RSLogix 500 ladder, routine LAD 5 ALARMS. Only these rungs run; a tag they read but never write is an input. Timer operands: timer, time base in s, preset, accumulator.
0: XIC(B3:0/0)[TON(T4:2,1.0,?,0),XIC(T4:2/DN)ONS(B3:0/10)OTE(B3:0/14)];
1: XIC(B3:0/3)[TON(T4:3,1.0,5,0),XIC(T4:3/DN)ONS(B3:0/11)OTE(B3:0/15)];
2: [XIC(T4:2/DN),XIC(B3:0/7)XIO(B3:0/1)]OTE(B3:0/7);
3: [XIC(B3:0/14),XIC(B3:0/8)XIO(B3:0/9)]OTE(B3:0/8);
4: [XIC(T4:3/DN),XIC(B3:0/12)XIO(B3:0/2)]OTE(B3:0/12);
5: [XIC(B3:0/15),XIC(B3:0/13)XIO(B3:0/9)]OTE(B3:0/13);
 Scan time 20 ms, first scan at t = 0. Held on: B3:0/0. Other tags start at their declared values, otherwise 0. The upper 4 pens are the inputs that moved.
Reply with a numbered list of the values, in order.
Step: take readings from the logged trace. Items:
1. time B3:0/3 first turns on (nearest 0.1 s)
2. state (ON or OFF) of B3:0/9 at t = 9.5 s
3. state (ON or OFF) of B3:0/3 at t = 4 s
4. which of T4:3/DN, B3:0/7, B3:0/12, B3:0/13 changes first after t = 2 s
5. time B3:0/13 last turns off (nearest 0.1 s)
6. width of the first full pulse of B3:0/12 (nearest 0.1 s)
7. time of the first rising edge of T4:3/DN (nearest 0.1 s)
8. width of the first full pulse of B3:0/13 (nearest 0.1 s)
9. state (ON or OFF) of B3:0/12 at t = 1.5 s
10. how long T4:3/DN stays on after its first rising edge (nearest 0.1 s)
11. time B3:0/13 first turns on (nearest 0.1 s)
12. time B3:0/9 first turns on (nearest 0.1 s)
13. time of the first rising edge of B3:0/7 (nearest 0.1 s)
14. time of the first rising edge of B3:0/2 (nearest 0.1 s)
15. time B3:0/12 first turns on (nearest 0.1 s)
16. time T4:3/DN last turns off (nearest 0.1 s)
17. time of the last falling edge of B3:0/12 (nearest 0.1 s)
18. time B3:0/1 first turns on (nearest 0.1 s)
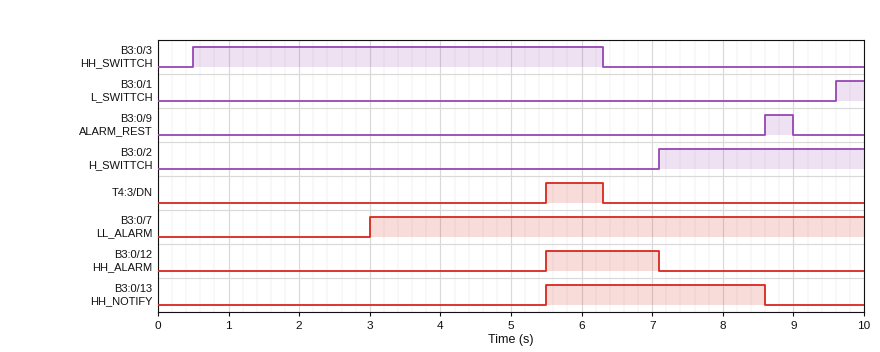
1. 0.5 s
2. OFF
3. ON
4. B3:0/7
5. 8.6 s
6. 1.6 s
7. 5.5 s
8. 3.1 s
9. OFF
10. 0.8 s
11. 5.5 s
12. 8.6 s
13. 3.0 s
14. 7.1 s
15. 5.5 s
16. 6.3 s
17. 7.1 s
18. 9.6 s
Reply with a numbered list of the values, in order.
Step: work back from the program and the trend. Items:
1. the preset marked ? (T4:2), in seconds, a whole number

1. 3 s
